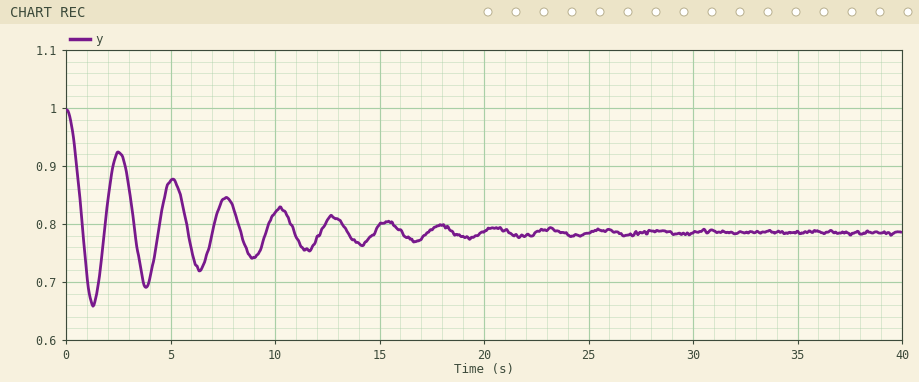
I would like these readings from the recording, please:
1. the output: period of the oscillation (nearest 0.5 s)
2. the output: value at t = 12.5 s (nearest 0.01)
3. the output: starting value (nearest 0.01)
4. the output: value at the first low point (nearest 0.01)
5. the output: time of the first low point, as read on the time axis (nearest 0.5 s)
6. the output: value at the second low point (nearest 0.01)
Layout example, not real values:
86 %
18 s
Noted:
2.5 s
0.81
1.00
0.66
1.5 s
0.69
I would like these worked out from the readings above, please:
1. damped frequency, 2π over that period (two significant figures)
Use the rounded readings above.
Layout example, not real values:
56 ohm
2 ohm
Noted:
2.5 rad/s
